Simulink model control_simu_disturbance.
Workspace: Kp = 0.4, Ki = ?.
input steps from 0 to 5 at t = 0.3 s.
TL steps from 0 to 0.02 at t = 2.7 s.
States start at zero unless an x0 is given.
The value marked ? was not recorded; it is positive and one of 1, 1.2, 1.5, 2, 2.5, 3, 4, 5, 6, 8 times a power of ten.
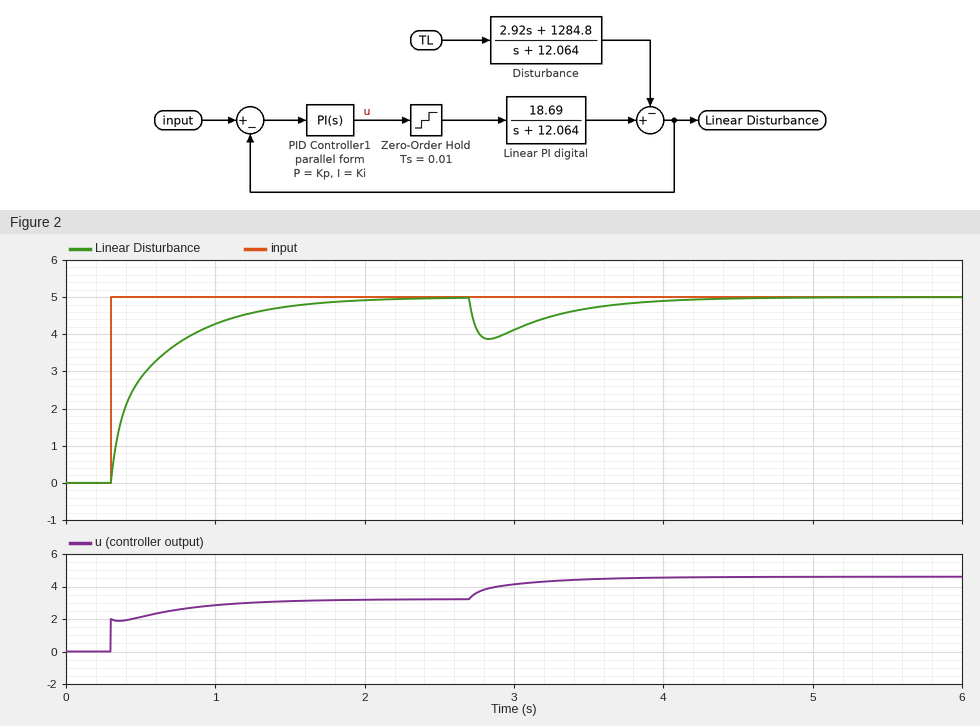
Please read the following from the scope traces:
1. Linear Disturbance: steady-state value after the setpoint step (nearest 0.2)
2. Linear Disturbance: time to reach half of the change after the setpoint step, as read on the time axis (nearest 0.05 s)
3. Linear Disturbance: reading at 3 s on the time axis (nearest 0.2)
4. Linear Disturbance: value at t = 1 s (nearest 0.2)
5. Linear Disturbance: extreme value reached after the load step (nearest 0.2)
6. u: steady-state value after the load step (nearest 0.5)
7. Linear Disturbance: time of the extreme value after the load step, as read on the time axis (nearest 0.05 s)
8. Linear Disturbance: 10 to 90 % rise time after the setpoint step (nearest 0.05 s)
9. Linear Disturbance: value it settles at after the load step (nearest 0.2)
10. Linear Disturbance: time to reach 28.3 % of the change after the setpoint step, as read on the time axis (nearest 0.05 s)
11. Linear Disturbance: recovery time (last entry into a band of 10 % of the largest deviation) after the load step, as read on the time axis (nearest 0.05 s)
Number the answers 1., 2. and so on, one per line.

1. 5.0
2. 0.45 s
3. 4.2
4. 4.2
5. 3.8
6. 4.5
7. 2.85 s
8. 0.85 s
9. 5.0
10. 0.35 s
11. 3.95 s
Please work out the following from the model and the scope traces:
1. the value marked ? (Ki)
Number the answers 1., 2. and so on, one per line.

1. 2
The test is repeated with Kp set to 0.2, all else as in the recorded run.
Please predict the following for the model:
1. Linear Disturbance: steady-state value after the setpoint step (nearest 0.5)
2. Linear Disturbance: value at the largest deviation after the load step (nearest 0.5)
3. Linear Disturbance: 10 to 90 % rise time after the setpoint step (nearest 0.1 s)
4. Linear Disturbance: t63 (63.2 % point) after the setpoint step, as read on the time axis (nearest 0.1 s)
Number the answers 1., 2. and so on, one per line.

1. 5.0
2. 3.5
3. 0.7 s
4. 0.6 s
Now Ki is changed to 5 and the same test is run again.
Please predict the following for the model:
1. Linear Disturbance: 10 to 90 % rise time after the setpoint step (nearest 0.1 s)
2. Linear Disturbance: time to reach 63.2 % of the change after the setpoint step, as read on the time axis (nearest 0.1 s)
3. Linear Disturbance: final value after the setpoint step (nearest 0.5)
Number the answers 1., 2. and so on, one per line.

1. 0.3 s
2. 0.4 s
3. 5.0
